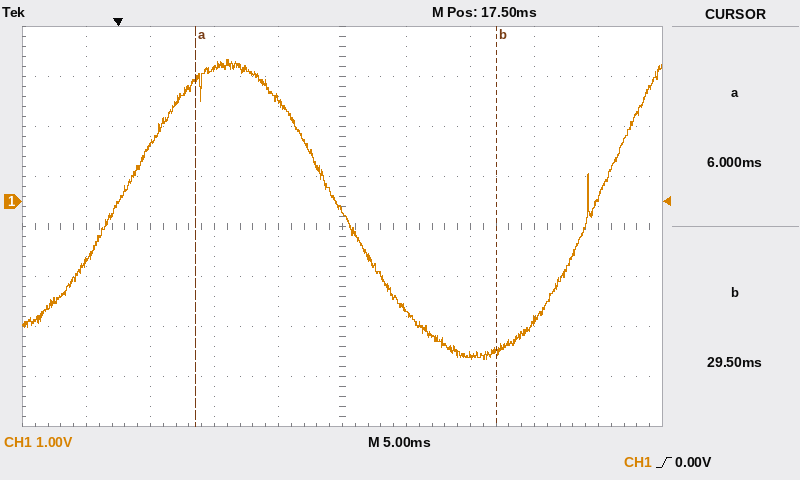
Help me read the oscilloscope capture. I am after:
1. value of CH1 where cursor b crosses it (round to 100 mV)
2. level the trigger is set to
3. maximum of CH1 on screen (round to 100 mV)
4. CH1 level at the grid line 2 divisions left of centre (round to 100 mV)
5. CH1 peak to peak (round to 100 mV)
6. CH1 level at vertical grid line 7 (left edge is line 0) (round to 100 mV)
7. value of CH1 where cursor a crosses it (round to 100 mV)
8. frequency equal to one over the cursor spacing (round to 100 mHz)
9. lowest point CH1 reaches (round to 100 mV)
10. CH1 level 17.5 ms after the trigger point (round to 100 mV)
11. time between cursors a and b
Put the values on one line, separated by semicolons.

-3.0 V; 0.00 V; 2.8 V; 2.7 V; 6.0 V; -3.1 V; 2.5 V; 42.6 Hz; -3.2 V; -200 mV; 23.5 ms
